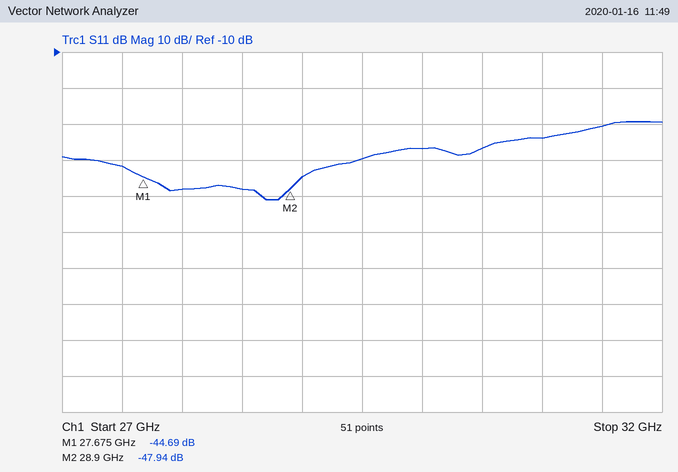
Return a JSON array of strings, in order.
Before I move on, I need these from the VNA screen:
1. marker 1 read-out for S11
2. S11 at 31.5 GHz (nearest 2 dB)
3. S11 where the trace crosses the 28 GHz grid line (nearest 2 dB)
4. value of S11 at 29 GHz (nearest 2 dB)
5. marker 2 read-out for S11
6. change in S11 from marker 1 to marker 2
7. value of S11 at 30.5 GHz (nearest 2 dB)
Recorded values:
["-44.69 dB", "-30 dB", "-48 dB", "-44 dB", "-47.94 dB", "-3.25 dB", "-36 dB"]
